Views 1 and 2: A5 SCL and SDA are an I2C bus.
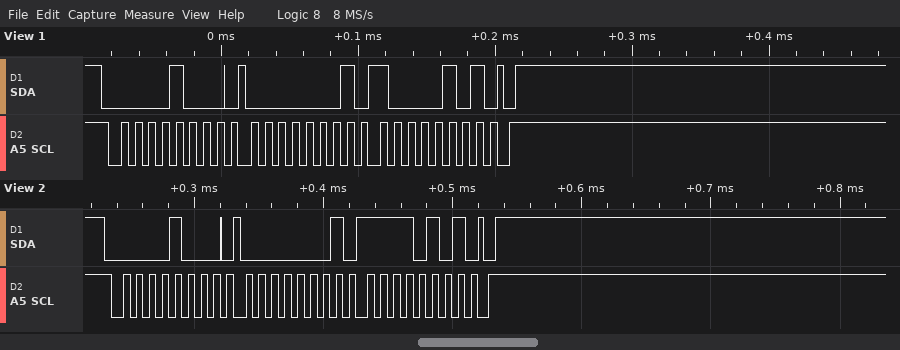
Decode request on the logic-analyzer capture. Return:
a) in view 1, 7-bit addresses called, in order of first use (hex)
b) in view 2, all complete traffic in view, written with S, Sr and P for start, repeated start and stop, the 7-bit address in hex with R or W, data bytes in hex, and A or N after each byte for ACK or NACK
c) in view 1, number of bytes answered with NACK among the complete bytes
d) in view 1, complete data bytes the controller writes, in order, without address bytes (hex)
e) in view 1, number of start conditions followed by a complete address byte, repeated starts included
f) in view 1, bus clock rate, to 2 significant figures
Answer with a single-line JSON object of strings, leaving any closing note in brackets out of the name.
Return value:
{"in view 1, 7-bit addresses called, in order of first use": "0x04", "in view 2, all complete traffic in view, written with S, Sr and P for start, repeated start and stop, the 7-bit address in hex with R or W, data bytes in hex, and A or N after each byte for ACK or NACK": "S 04W A 01 A F5 A P", "in view 1, number of bytes answered with NACK among the complete bytes": "0", "in view 1, complete data bytes the controller writes, in order, without address bytes": "01 85", "in view 1, number of start conditions followed by a complete address byte, repeated starts included": "1", "in view 1, bus clock rate, to 2 significant figures": "100 kHz"}
